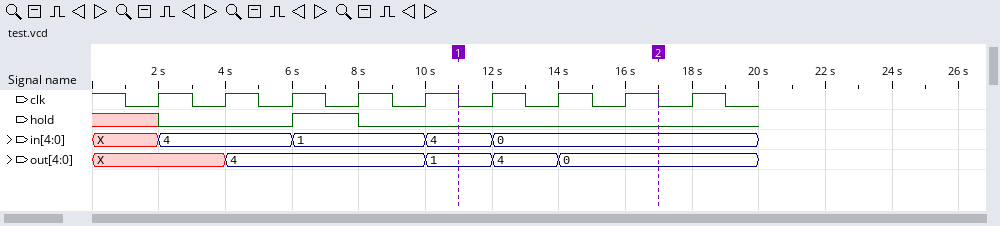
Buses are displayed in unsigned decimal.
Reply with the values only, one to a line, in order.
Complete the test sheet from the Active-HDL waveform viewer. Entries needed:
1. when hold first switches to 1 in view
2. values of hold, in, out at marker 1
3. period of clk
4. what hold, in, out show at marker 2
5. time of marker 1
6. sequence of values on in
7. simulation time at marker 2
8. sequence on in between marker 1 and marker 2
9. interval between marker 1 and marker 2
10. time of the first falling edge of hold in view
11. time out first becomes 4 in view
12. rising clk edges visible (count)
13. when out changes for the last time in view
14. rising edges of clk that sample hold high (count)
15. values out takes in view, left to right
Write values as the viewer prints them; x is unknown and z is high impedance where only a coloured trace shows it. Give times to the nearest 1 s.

6 s
hold=0, in=4, out=1
2 s
hold=0, in=0, out=0
11 s
X, 4, 1, 4, 0
17 s
4, 0
6 s
8 s
4 s
9
14 s
1
X, 4, 1, 4, 0
